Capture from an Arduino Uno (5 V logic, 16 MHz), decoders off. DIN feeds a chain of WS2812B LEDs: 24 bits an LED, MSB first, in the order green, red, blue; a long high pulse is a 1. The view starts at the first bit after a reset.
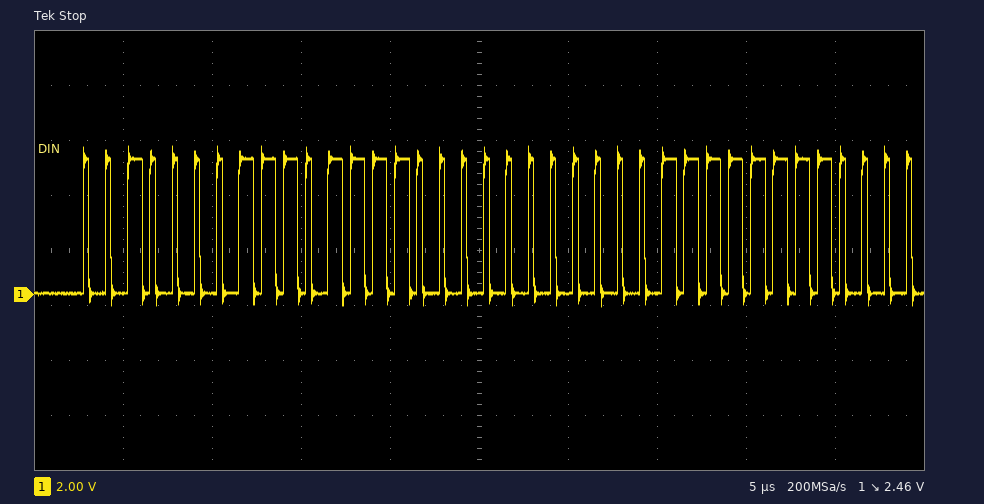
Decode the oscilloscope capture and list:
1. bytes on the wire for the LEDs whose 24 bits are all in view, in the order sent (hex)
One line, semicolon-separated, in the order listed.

21 DE 00
